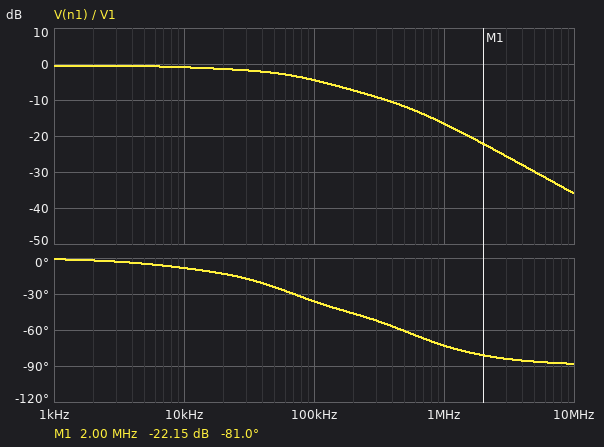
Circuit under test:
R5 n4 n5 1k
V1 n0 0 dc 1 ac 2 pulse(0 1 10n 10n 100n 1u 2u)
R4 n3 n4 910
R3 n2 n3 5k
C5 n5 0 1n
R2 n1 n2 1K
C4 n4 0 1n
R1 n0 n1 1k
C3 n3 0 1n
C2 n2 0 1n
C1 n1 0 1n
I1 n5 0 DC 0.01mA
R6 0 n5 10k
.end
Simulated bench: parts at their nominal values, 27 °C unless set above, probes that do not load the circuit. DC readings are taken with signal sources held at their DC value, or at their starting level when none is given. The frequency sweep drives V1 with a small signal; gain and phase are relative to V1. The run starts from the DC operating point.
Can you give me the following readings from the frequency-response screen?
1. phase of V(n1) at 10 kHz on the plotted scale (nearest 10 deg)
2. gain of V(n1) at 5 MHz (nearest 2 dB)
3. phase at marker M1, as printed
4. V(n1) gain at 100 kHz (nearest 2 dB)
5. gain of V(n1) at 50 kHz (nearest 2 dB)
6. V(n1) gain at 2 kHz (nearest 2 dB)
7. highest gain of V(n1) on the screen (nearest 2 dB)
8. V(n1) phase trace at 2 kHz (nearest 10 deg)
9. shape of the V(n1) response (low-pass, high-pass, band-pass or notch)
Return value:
-10 deg
-30 dB
-81.0 deg
-4 dB
-2 dB
0 dB
0 dB
0 deg
low-pass
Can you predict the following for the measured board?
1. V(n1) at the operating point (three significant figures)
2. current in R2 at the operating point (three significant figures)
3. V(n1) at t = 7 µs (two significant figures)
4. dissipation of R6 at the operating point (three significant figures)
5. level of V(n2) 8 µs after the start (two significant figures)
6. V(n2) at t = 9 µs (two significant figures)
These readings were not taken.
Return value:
942 mV
58.2 µA
630 mV
23.2 µW
360 mV
430 mV
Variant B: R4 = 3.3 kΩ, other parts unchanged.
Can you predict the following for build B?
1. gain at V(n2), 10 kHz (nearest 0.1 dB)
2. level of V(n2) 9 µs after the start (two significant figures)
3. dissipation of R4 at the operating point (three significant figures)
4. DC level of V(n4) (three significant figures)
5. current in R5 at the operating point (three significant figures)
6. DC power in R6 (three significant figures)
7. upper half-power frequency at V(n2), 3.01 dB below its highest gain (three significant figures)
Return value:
-1.6 dB
440 mV
8.80 µW
468 mV
51.6 µA
17.3 µW
45.5 kHz
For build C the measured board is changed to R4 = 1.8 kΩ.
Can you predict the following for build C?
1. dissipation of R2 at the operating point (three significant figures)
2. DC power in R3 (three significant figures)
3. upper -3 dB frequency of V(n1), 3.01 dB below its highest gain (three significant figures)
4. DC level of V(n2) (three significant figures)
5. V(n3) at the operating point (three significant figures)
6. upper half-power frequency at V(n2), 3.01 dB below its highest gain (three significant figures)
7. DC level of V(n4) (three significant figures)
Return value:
3.09 µW
15.4 µW
73.4 kHz
889 mV
611 mV
45.4 kHz
511 mV
